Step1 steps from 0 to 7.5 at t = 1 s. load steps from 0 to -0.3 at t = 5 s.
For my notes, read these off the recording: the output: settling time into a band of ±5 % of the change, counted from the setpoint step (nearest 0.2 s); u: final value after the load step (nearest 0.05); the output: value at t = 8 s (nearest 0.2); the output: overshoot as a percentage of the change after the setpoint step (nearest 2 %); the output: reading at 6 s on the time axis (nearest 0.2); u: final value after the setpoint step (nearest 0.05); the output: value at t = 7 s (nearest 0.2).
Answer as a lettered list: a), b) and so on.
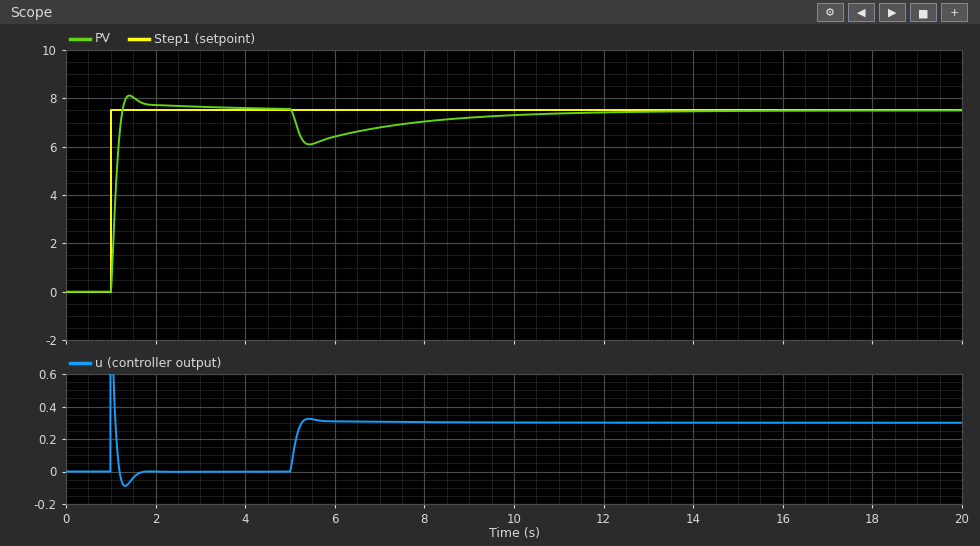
a) 0.6 s
b) 0.30
c) 7.0
d) 8 %
e) 6.4
f) 0.00
g) 6.8
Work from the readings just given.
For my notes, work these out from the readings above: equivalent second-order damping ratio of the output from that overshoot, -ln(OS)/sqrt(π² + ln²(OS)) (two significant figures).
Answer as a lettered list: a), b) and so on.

a) 0.63
